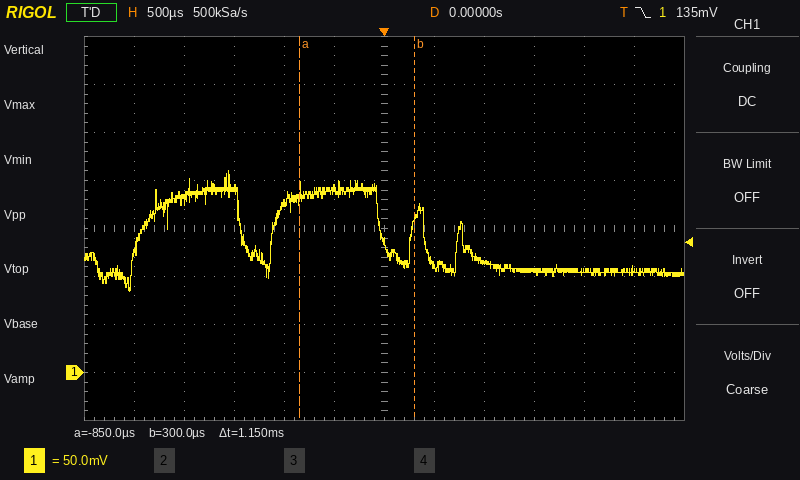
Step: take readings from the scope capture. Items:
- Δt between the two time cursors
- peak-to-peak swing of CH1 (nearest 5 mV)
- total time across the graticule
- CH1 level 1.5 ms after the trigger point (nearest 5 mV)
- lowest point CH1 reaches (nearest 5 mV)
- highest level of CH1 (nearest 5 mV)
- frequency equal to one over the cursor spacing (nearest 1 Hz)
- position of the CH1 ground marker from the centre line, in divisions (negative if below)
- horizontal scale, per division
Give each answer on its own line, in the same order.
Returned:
1.15 ms
125 mV
6 ms
105 mV
85 mV
210 mV
870 Hz
-3.0 div
500 µs
